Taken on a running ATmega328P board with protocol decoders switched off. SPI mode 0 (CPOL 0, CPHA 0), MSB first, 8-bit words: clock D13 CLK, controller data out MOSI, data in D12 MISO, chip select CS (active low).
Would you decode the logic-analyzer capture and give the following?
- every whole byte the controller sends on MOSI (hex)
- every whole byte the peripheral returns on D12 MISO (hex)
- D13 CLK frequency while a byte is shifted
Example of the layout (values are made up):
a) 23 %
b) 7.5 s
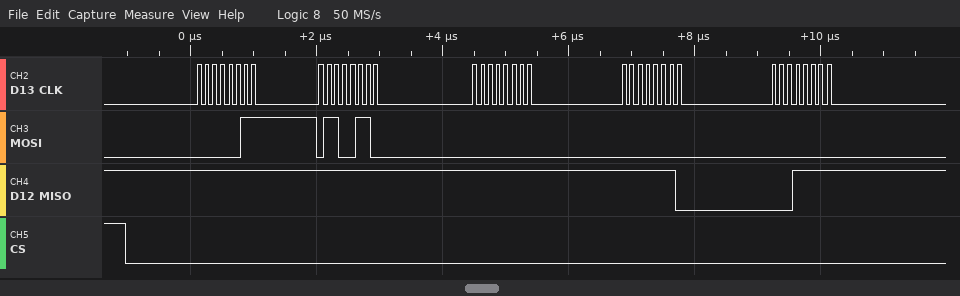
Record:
a) 03 66 00 00 00
b) FF FF FF FE 1F
c) 8 MHz
